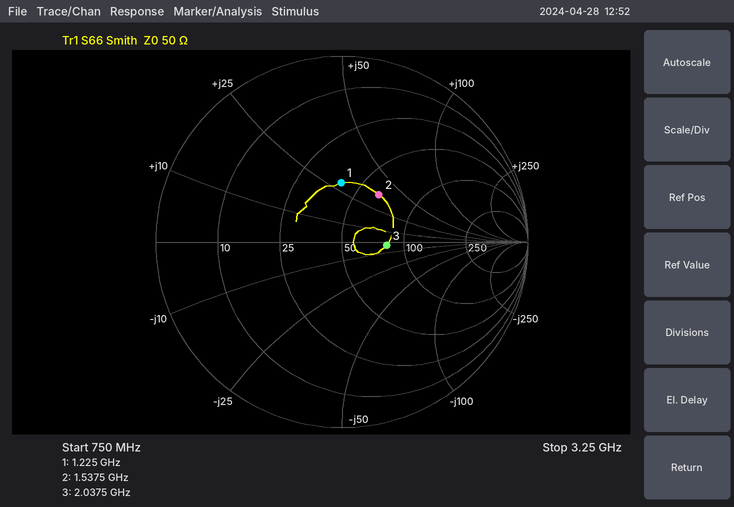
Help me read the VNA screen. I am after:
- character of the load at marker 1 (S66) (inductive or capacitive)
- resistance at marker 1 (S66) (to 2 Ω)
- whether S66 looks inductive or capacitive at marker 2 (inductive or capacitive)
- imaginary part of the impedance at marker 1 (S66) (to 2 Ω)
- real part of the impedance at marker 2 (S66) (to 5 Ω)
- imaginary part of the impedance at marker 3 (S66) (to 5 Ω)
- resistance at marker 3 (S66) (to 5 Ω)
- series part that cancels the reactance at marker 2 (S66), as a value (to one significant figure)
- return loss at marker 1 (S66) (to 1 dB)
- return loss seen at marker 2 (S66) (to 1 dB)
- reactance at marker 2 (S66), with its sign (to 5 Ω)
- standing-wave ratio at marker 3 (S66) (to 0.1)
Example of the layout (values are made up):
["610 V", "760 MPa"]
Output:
["inductive", "40 Ω", "inductive", "+28 Ω", "65 Ω", "-5 Ω", "80 Ω", "3 pF", "10 dB", "10 dB", "+35 Ω", "1.6"]
